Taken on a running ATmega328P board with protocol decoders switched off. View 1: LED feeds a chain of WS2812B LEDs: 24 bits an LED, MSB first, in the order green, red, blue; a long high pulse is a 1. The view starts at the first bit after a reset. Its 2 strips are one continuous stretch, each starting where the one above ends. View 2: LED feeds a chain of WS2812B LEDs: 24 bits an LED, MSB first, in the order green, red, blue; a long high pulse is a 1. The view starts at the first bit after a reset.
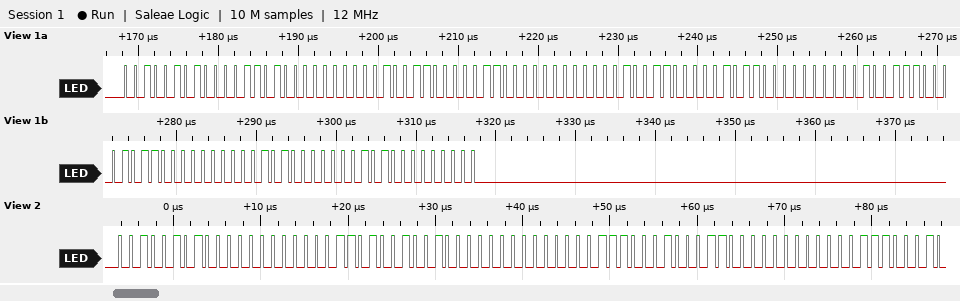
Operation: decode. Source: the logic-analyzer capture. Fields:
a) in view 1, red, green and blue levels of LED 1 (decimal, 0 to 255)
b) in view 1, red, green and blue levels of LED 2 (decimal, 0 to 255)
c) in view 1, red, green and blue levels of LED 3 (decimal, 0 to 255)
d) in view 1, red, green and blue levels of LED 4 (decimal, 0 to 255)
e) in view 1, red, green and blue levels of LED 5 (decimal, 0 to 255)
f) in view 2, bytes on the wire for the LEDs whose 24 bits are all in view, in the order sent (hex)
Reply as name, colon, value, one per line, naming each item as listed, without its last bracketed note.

in view 1, red, green and blue levels of LED 1: 13, 37, 0
in view 1, red, green and blue levels of LED 2: 12, 38, 0
in view 1, red, green and blue levels of LED 3: 11, 38, 0
in view 1, red, green and blue levels of LED 4: 11, 39, 0
in view 1, red, green and blue levels of LED 5: 10, 40, 0
in view 2, bytes on the wire for the LEDs whose 24 bits are all in view, in the order sent: 25 00 0D 24 00 0E 23 00 0E
